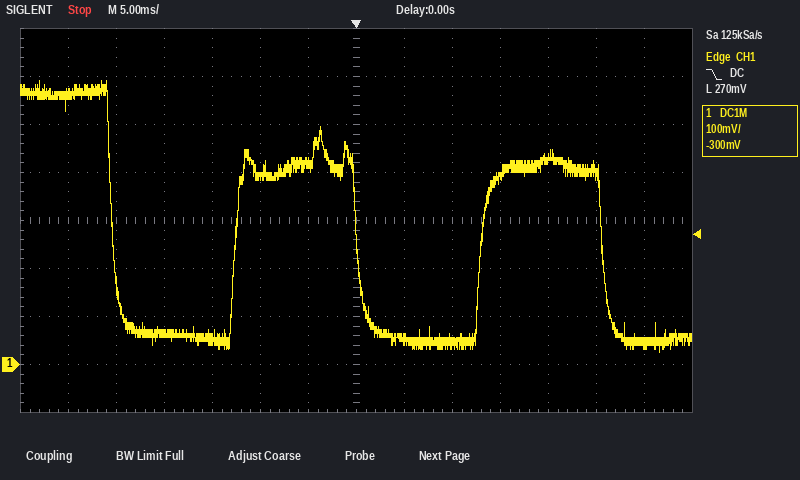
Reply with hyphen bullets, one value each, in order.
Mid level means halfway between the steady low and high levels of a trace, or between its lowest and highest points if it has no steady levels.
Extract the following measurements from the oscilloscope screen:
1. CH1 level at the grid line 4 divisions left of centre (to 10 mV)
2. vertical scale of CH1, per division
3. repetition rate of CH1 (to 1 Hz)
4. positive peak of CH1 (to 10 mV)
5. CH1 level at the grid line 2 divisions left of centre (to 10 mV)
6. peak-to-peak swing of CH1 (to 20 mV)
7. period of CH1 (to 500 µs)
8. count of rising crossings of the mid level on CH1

- 60 mV
- 100 mV
- 39 Hz
- 590 mV
- 390 mV
- 560 mV
- 25.5 ms
- 2
